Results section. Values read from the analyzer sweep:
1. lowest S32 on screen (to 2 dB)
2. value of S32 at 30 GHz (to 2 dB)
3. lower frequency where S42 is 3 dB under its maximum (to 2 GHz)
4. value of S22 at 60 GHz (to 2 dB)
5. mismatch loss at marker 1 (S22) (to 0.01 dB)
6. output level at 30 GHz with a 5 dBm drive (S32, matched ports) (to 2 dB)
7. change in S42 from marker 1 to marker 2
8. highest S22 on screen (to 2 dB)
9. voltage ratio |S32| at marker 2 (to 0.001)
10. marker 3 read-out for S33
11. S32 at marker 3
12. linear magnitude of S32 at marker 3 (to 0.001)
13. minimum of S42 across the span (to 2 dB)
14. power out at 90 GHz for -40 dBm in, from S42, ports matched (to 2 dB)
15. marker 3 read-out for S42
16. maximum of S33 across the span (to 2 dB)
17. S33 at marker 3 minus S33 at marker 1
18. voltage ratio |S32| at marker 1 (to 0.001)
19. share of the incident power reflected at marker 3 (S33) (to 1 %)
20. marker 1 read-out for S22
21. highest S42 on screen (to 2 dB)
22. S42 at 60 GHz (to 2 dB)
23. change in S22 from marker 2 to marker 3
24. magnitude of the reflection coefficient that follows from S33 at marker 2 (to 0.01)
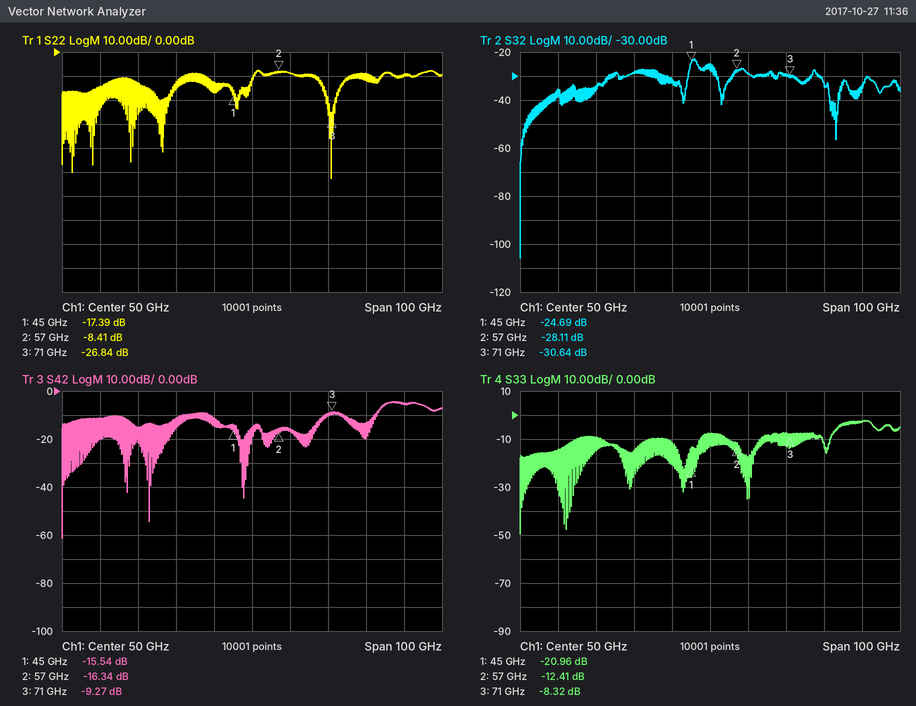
-106 dB
-28 dB
84 GHz
-8 dB
0.08 dB
-24 dBm
-0.80 dB
-8 dB
0.039
-8.32 dB
-30.64 dB
0.029
-62 dB
-46 dBm
-9.27 dB
-2 dB
12.64 dB
0.058
15 %
-17.39 dB
-4 dB
-16 dB
-18.43 dB
0.24
